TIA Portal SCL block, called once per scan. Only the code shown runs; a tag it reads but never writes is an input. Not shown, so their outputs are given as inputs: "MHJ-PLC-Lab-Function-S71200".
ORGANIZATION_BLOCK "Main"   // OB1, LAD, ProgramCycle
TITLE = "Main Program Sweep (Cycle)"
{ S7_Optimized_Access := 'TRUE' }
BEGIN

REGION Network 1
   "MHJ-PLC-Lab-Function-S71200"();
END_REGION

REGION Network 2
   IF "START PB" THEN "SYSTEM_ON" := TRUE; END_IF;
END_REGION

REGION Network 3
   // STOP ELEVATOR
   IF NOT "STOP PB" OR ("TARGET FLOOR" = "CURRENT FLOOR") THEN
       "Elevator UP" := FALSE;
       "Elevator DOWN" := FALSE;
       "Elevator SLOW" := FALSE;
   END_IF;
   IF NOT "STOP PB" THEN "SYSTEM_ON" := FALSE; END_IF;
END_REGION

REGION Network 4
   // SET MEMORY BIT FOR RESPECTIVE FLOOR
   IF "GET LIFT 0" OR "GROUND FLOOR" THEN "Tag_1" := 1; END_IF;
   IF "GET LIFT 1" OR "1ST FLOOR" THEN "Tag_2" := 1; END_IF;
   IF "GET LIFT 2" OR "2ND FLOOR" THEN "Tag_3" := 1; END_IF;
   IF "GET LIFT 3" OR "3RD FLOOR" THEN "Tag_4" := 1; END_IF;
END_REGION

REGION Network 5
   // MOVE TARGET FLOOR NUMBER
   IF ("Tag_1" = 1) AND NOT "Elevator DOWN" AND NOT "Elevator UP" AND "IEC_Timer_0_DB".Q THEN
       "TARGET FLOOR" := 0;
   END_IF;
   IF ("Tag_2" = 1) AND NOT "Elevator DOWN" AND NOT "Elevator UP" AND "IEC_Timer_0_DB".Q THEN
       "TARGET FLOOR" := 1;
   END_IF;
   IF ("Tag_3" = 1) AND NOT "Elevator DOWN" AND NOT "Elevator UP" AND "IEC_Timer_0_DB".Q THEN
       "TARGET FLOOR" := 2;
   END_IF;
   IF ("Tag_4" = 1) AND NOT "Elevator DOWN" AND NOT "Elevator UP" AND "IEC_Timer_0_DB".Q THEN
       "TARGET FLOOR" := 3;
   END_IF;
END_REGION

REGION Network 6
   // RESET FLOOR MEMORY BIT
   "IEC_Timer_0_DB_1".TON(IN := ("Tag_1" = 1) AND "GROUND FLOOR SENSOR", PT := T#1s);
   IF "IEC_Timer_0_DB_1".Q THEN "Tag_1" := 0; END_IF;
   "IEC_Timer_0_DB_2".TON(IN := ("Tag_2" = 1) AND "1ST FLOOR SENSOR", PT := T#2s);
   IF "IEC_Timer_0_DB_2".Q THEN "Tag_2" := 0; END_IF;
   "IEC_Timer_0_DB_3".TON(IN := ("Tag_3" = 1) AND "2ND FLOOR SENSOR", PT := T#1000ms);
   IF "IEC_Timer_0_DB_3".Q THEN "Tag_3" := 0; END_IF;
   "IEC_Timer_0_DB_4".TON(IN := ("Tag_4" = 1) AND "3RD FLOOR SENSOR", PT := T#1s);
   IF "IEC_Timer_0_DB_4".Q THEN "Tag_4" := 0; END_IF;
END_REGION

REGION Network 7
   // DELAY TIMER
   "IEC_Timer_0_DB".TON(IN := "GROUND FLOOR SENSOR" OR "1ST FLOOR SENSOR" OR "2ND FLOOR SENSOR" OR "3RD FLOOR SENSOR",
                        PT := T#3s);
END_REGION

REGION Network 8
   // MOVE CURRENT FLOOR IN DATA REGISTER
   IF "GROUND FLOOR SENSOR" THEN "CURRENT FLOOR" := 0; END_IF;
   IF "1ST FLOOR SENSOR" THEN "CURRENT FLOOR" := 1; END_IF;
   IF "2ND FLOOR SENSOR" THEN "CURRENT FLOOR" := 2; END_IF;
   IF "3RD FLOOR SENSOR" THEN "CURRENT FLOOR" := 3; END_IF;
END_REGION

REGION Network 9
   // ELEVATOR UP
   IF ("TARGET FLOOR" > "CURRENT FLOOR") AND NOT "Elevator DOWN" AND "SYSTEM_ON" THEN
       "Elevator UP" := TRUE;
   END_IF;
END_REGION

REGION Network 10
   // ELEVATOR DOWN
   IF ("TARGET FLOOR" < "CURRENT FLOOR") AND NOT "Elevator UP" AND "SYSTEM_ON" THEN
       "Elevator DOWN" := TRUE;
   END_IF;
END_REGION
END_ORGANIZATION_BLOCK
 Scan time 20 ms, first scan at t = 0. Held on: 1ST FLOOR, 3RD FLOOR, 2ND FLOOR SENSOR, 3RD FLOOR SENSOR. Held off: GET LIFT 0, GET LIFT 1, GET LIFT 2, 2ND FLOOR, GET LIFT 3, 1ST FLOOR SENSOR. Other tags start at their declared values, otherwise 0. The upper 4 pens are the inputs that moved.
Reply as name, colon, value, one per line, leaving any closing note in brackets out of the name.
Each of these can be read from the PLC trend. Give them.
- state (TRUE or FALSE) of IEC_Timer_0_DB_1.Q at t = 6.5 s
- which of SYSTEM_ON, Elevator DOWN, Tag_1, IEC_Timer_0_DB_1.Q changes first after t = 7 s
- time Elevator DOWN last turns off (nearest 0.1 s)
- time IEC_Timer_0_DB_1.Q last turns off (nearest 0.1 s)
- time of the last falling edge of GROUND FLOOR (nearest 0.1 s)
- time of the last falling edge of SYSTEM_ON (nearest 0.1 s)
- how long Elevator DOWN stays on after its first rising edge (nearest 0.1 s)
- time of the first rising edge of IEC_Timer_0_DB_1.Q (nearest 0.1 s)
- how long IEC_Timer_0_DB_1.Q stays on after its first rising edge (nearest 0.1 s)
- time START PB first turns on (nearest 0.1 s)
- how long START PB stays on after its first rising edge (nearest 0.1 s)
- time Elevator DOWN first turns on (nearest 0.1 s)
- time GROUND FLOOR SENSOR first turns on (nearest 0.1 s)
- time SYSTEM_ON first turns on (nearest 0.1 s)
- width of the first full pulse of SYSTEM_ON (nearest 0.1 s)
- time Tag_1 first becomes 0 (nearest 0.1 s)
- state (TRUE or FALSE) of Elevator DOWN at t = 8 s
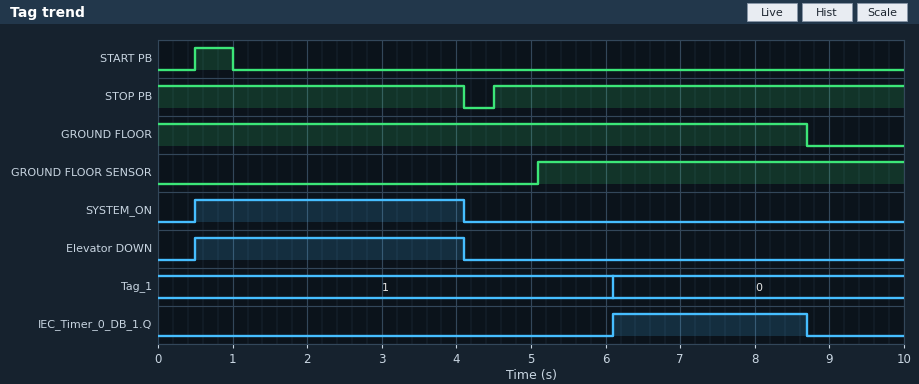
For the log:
state (TRUE or FALSE) of IEC_Timer_0_DB_1.Q at t = 6.5 s: TRUE
which of SYSTEM_ON, Elevator DOWN, Tag_1, IEC_Timer_0_DB_1.Q changes first after t = 7 s: IEC_Timer_0_DB_1.Q
time Elevator DOWN last turns off: 4.1 s
time IEC_Timer_0_DB_1.Q last turns off: 8.7 s
time of the last falling edge of GROUND FLOOR: 8.7 s
time of the last falling edge of SYSTEM_ON: 4.1 s
how long Elevator DOWN stays on after its first rising edge: 3.6 s
time of the first rising edge of IEC_Timer_0_DB_1.Q: 6.1 s
how long IEC_Timer_0_DB_1.Q stays on after its first rising edge: 2.6 s
time START PB first turns on: 0.5 s
how long START PB stays on after its first rising edge: 0.5 s
time Elevator DOWN first turns on: 0.5 s
time GROUND FLOOR SENSOR first turns on: 5.1 s
time SYSTEM_ON first turns on: 0.5 s
width of the first full pulse of SYSTEM_ON: 3.6 s
time Tag_1 first becomes 0: 6.1 s
state (TRUE or FALSE) of Elevator DOWN at t = 8 s: FALSE
